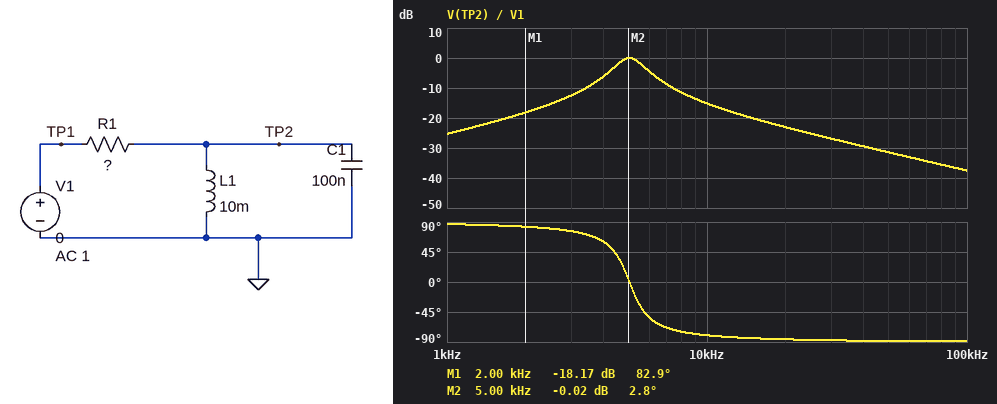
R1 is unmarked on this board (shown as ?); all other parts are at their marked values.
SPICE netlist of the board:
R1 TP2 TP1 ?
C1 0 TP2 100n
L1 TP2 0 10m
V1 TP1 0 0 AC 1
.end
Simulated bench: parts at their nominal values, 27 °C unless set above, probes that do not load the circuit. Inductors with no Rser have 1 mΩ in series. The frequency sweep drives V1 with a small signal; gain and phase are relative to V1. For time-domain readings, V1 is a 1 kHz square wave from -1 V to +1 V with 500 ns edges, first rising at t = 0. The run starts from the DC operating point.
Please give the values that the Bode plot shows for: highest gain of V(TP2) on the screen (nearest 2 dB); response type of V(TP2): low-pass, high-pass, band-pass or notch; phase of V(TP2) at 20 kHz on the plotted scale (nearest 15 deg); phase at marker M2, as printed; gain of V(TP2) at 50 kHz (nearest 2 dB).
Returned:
0 dB
band-pass
-90 deg
2.8 deg
-32 dB
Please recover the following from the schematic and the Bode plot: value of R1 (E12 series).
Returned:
1.2 kΩ
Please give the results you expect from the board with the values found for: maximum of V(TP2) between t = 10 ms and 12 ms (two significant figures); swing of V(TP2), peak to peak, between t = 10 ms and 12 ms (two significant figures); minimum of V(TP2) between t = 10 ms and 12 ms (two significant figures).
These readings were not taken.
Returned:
500 mV
990 mV
-500 mV
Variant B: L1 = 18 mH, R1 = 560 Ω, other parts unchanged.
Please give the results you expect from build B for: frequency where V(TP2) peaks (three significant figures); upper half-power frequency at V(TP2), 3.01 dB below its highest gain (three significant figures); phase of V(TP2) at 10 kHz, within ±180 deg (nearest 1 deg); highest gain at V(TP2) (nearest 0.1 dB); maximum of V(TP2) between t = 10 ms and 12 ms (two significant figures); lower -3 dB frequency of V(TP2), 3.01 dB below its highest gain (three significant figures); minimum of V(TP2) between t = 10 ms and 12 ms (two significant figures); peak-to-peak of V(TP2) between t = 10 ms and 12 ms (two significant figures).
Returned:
3.75 kHz
5.43 kHz
-72 deg
0 dB
940 mV
2.59 kHz
-940 mV
1.9 V
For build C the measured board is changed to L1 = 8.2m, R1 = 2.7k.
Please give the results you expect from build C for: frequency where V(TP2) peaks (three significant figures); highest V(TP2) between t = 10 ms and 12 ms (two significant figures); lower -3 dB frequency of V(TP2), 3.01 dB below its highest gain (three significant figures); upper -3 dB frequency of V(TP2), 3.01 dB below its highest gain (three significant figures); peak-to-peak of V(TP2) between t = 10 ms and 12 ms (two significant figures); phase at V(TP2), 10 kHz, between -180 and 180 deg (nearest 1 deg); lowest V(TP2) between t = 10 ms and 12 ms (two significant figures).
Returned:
5.56 kHz
180 mV
5.27 kHz
5.86 kHz
350 mV
-85 deg
-180 mV
